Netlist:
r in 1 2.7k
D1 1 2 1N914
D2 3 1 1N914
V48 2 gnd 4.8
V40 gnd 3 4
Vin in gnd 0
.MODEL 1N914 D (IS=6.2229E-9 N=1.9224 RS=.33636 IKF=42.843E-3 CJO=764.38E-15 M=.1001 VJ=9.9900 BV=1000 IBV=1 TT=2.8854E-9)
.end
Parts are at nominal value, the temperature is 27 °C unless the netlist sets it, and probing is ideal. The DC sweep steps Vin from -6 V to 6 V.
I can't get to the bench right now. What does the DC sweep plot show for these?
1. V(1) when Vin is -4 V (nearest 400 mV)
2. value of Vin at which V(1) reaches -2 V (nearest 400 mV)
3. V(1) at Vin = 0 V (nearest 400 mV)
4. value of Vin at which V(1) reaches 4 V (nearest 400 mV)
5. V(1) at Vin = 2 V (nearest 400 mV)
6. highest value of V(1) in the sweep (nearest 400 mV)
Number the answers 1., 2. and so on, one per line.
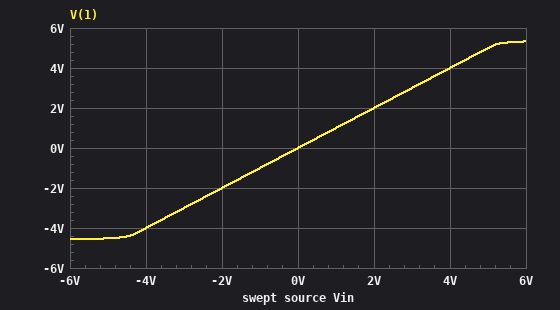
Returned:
1. -4.0 V
2. -2.0 V
3. 0 V
4. 4.0 V
5. 2.0 V
6. 5.2 V
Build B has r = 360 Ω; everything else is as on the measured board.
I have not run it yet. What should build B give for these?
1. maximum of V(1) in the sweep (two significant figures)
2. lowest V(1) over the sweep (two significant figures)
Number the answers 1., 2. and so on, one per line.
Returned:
1. 5.4 V
2. -4.7 V
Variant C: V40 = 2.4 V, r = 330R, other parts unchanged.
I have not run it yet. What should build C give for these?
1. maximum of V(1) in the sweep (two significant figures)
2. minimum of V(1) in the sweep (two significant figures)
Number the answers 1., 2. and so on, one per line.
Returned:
1. 5.4 V
2. -3.1 V
